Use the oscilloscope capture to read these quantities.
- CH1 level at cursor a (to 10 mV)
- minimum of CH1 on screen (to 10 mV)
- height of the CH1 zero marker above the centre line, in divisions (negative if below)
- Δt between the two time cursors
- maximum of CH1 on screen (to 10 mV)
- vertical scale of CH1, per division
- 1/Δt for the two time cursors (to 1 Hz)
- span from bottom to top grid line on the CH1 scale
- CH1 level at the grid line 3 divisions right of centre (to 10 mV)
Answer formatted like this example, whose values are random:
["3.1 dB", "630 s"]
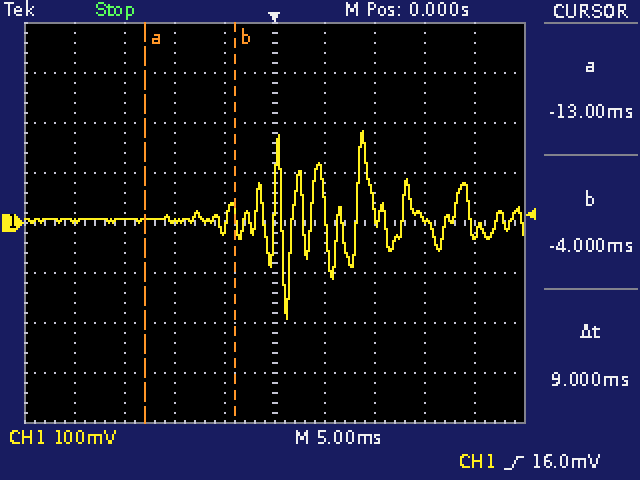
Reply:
["0 mV", "-190 mV", "0.0 div", "9 ms", "180 mV", "100 mV", "111 Hz", "800 mV", "10 mV"]
